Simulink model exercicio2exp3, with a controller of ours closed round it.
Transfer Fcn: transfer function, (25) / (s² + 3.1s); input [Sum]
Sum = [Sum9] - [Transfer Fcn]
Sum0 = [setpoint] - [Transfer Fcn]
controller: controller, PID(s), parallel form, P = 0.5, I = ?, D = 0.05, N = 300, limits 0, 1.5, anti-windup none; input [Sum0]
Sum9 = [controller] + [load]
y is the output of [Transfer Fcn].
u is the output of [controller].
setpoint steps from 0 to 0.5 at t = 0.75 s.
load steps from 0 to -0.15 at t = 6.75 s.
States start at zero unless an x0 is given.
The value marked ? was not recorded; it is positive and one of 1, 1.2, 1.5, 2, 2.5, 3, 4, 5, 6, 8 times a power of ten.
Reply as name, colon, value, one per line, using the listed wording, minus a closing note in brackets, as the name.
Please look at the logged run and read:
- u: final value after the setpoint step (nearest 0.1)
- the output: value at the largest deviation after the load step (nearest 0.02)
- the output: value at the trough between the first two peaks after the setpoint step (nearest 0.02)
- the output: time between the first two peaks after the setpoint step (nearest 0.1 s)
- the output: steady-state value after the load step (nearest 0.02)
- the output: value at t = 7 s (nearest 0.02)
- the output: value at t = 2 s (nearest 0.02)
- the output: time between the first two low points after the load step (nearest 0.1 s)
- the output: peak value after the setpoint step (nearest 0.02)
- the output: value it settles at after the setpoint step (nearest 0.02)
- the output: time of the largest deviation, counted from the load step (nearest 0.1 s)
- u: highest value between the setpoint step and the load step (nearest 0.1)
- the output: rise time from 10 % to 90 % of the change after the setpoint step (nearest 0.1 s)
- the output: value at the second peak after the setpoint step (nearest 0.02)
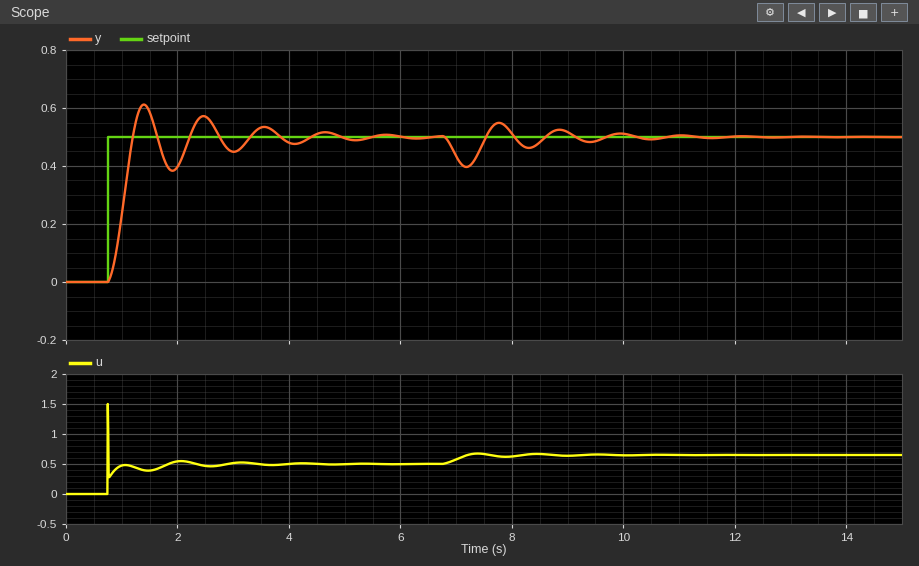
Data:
u: final value after the setpoint step: 0.5
the output: value at the largest deviation after the load step: 0.40
the output: value at the trough between the first two peaks after the setpoint step: 0.38
the output: time between the first two peaks after the setpoint step: 1.1 s
the output: steady-state value after the load step: 0.50
the output: value at t = 7 s: 0.44
the output: value at t = 2 s: 0.40
the output: time between the first two low points after the load step: 1.1 s
the output: peak value after the setpoint step: 0.62
the output: value it settles at after the setpoint step: 0.50
the output: time of the largest deviation, counted from the load step: 0.4 s
u: highest value between the setpoint step and the load step: 1.5
the output: rise time from 10 % to 90 % of the change after the setpoint step: 0.3 s
the output: value at the second peak after the setpoint step: 0.58
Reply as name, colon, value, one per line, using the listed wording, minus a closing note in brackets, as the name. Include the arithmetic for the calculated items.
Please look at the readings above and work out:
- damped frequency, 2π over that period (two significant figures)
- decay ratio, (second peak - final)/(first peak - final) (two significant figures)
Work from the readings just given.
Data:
damped frequency, 2π over that period: 2π / 1.1 = 5.7 rad/s
decay ratio, (second peak - final)/(first peak - final): (0.58 - 0.5) / (0.62 - 0.5) = 0.67
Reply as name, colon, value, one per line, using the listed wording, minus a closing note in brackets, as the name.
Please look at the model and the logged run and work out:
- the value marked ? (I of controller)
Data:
the value marked ?: 4
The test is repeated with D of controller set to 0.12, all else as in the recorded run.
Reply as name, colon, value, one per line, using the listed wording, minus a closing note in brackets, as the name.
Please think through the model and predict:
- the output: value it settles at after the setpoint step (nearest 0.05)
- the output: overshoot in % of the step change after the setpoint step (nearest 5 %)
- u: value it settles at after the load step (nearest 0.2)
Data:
the output: value it settles at after the setpoint step: 0.50
the output: overshoot in % of the step change after the setpoint step: 15 %
u: value it settles at after the load step: 0.6
